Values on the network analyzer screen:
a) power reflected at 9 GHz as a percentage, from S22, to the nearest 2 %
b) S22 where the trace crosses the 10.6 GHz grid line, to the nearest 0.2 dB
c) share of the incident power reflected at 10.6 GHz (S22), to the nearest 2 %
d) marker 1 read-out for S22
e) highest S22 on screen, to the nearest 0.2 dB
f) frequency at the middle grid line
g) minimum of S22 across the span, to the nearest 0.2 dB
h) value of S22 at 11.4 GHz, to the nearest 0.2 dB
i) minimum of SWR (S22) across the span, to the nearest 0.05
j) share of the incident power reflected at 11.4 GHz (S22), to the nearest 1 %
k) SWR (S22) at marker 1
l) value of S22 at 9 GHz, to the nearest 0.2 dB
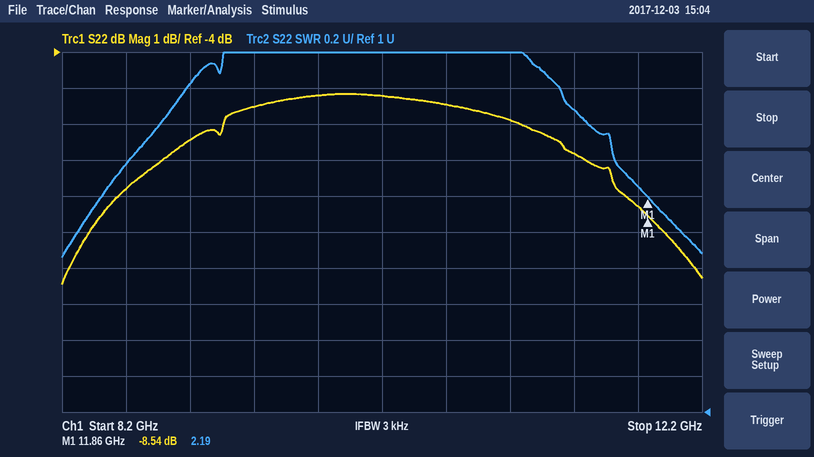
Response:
22 %
-5.4 dB
28 %
-8.54 dB
-5.2 dB
10.2 GHz
-10.4 dB
-6.8 dB
1.85
21 %
2.19
-6.4 dB
